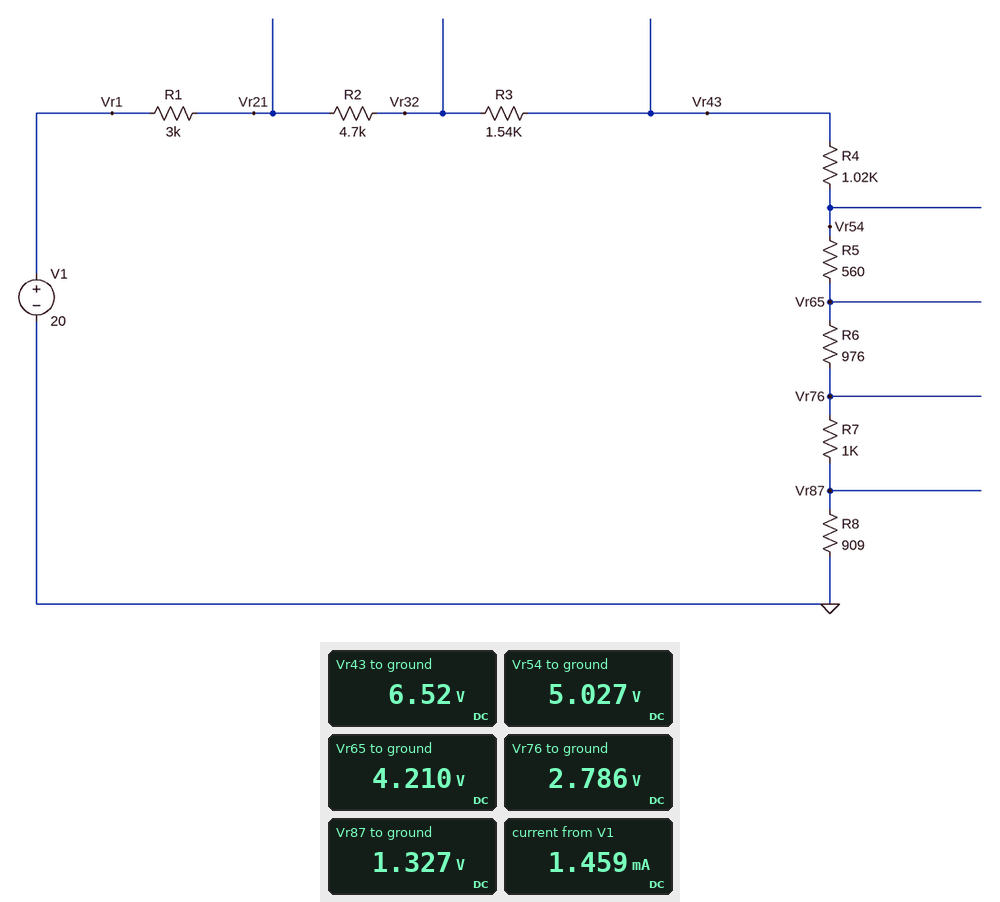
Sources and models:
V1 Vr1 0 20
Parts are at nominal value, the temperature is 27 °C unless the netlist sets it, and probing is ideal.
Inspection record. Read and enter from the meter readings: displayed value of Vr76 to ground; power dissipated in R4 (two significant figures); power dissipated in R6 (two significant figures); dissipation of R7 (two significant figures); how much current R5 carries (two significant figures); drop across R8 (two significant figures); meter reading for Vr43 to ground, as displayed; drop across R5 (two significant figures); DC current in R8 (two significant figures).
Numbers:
2.786 V
2.2 mW
2.1 mW
2.1 mW
1.5 mA
1.3 V
6.52 V
820 mV
1.5 mA
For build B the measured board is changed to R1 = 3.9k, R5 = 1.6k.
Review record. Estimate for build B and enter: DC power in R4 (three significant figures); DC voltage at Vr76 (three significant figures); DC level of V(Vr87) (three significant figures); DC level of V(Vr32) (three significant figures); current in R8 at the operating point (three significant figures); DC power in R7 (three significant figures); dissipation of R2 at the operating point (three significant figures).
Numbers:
1.67 mW
2.44 V
1.16 V
9.01 V
1.28 mA
1.63 mW
7.68 mW
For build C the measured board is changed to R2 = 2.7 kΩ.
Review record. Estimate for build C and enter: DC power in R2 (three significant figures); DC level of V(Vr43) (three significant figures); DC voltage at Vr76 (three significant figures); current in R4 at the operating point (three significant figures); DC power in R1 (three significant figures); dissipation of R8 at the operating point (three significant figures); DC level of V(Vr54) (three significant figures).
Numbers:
7.88 mW
7.63 V
3.26 V
1.71 mA
8.76 mW
2.65 mW
5.89 V
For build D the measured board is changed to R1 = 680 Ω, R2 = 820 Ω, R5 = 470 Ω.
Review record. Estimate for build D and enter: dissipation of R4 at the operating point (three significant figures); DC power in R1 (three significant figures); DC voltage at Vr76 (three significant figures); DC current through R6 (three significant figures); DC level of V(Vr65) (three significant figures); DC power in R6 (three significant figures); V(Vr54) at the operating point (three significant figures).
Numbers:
7.42 mW
4.95 mW
5.15 V
2.70 mA
7.78 V
7.10 mW
9.05 V
